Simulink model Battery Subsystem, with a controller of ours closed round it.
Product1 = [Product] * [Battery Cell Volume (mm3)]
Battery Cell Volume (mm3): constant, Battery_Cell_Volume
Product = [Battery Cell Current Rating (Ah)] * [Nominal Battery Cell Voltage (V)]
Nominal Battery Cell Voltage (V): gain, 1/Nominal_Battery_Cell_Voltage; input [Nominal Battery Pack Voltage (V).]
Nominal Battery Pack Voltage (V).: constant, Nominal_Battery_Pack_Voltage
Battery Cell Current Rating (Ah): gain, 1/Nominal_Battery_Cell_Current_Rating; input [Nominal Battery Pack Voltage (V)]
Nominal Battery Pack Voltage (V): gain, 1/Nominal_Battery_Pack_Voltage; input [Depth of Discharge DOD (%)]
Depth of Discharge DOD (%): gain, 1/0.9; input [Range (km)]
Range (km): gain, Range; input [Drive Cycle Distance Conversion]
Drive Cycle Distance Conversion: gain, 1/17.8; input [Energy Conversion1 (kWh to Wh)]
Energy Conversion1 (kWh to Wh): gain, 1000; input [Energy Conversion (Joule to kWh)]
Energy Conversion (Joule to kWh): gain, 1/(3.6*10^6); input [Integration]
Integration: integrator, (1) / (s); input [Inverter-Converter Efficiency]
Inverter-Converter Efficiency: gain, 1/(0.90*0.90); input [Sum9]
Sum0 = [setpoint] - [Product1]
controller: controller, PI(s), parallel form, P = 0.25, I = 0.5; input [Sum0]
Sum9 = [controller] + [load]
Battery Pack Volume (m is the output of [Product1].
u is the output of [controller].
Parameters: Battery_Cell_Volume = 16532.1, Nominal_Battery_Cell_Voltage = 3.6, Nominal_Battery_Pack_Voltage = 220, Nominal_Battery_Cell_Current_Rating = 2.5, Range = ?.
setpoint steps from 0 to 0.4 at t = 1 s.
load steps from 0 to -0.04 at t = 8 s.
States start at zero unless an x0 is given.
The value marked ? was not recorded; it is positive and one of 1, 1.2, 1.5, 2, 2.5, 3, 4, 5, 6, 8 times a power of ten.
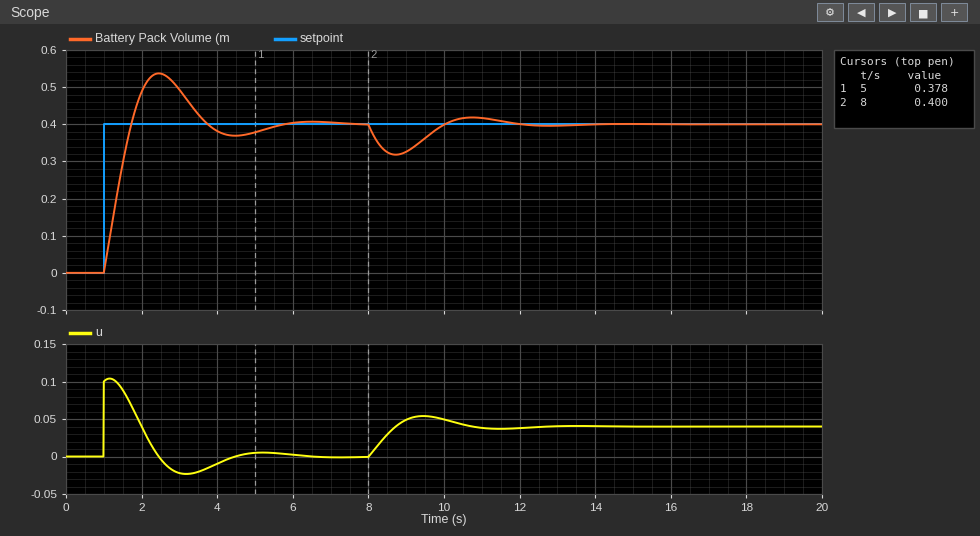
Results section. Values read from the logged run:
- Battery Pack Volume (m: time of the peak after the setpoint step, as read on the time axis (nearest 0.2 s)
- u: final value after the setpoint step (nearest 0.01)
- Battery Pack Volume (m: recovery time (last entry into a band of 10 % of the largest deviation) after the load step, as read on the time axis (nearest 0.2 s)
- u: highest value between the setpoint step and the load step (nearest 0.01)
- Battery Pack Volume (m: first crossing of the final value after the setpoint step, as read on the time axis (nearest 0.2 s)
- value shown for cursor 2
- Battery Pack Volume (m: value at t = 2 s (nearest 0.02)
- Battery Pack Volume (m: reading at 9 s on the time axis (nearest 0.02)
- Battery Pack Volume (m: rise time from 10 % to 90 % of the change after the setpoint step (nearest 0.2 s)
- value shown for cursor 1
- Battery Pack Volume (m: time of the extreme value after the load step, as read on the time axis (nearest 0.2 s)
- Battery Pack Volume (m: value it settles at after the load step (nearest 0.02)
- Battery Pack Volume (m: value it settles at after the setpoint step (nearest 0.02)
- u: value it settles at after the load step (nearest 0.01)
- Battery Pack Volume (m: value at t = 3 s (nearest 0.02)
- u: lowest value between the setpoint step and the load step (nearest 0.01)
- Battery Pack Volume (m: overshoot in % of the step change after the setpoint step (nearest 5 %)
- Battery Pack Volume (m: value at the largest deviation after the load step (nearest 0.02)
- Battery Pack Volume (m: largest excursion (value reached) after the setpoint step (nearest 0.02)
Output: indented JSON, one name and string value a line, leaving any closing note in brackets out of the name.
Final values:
{
  "Battery Pack Volume (m: time of the peak after the setpoint step, as read on the time axis": "2.4 s",
  "u: final value after the setpoint step": "0.00",
  "Battery Pack Volume (m: recovery time (last entry into a band of 10 % of the largest deviation) after the load step, as read on the time axis": "11.6 s",
  "u: highest value between the setpoint step and the load step": "0.10",
  "Battery Pack Volume (m: first crossing of the final value after the setpoint step, as read on the time axis": "1.8 s",
  "value shown for cursor 2": "0.400",
  "Battery Pack Volume (m: value at t = 2 s": "0.48",
  "Battery Pack Volume (m: reading at 9 s on the time axis": "0.32",
  "Battery Pack Volume (m: rise time from 10 % to 90 % of the change after the setpoint step": "0.6 s",
  "value shown for cursor 1": "0.378",
  "Battery Pack Volume (m: time of the extreme value after the load step, as read on the time axis": "8.8 s",
  "Battery Pack Volume (m: value it settles at after the load step": "0.40",
  "Battery Pack Volume (m: value it settles at after the setpoint step": "0.40",
  "u: value it settles at after the load step": "0.04",
  "Battery Pack Volume (m: value at t = 3 s": "0.50",
  "u: lowest value between the setpoint step and the load step": "-0.02",
  "Battery Pack Volume (m: overshoot in % of the step change after the setpoint step": "35 %",
  "Battery Pack Volume (m: value at the largest deviation after the load step": "0.32",
  "Battery Pack Volume (m: largest excursion (value reached) after the setpoint step": "0.54"
}
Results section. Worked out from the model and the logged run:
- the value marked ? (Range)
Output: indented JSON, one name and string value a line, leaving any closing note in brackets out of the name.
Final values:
{
  "the value marked ?": "150"
}
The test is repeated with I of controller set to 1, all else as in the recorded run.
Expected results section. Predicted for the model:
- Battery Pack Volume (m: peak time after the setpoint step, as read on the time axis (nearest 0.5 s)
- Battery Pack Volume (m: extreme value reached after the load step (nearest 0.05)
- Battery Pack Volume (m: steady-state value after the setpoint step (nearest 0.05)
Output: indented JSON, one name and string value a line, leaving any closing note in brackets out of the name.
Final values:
{
  "Battery Pack Volume (m: peak time after the setpoint step, as read on the time axis": "2.0 s",
  "Battery Pack Volume (m: extreme value reached after the load step": "0.35",
  "Battery Pack Volume (m: steady-state value after the setpoint step": "0.40"
}
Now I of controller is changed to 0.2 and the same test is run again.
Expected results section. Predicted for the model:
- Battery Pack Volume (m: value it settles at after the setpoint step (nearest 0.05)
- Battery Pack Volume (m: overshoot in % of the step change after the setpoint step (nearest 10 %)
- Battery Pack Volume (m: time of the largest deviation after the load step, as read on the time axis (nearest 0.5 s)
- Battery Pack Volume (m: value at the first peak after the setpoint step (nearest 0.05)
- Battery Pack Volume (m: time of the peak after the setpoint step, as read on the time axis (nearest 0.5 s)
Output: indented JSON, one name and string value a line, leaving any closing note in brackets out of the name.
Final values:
{
  "Battery Pack Volume (m: value it settles at after the setpoint step": "0.40",
  "Battery Pack Volume (m: overshoot in % of the step change after the setpoint step": "20 %",
  "Battery Pack Volume (m: time of the largest deviation after the load step, as read on the time axis": "9.0 s",
  "Battery Pack Volume (m: value at the first peak after the setpoint step": "0.50",
  "Battery Pack Volume (m: time of the peak after the setpoint step, as read on the time axis": "3.0 s"
}
